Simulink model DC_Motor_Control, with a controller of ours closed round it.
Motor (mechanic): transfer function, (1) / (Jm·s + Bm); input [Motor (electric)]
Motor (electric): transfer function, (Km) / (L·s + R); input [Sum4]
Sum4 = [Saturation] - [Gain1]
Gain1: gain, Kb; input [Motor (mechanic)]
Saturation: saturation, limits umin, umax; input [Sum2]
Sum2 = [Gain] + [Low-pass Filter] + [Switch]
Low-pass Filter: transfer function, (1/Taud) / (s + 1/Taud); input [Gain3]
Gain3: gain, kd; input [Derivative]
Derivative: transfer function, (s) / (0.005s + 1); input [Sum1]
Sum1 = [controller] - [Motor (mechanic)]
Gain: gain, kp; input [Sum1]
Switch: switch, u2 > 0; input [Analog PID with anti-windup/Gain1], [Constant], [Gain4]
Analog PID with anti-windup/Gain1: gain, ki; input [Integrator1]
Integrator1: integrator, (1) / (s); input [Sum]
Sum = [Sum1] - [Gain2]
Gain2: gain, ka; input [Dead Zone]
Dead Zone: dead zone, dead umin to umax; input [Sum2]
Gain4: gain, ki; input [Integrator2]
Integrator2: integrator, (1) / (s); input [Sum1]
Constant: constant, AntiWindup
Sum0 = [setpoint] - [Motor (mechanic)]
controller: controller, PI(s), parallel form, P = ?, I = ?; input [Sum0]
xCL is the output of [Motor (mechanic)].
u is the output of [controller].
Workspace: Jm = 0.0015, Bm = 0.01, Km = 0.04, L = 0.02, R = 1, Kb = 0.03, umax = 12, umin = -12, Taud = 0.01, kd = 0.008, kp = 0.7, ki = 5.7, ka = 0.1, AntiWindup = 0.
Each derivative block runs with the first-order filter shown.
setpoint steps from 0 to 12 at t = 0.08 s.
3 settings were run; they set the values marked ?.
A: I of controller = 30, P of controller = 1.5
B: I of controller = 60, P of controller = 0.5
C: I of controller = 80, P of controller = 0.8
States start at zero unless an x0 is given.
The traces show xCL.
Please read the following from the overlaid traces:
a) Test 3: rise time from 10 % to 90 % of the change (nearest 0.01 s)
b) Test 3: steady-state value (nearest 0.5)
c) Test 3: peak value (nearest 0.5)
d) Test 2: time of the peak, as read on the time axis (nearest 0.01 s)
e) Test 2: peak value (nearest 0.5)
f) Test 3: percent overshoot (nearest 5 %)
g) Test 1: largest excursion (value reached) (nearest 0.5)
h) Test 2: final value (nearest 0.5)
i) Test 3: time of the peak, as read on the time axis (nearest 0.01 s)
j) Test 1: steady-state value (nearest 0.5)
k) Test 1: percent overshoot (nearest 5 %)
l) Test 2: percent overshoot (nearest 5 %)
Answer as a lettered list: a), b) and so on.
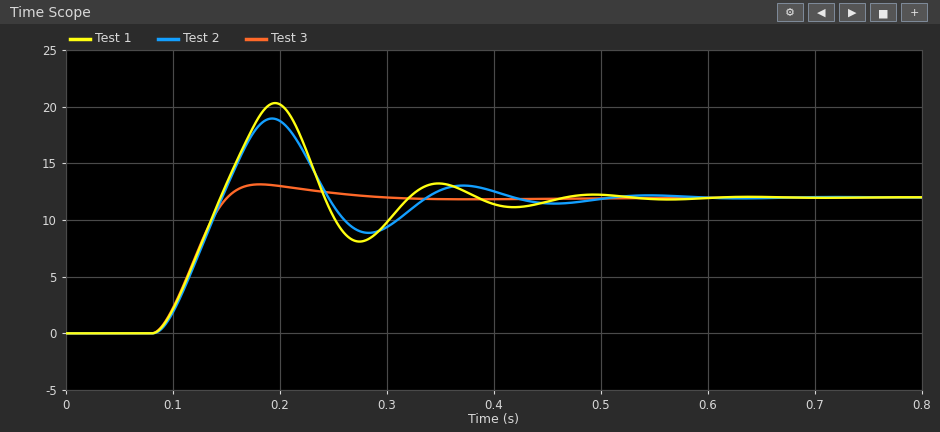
a) 0.05 s
b) 12.0
c) 13.0
d) 0.19 s
e) 19.0
f) 10 %
g) 20.5
h) 12.0
i) 0.18 s
j) 12.0
k) 70 %
l) 60 %
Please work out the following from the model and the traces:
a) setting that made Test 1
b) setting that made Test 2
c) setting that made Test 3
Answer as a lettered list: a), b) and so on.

a) C
b) B
c) A
